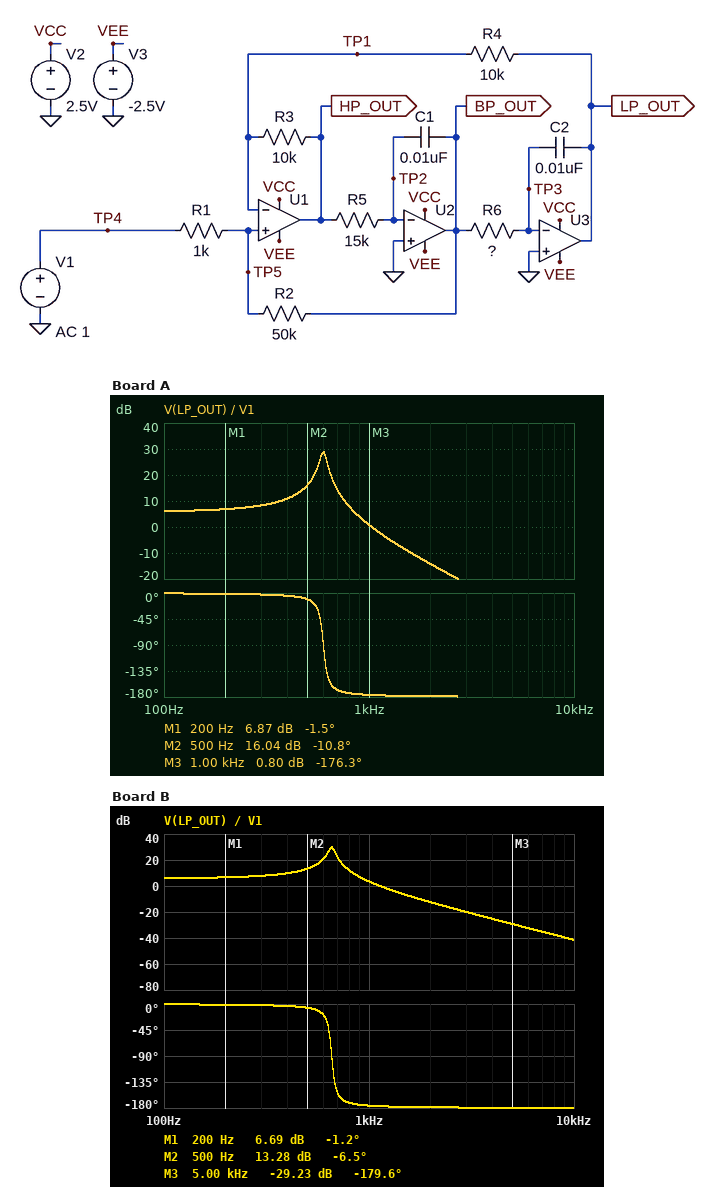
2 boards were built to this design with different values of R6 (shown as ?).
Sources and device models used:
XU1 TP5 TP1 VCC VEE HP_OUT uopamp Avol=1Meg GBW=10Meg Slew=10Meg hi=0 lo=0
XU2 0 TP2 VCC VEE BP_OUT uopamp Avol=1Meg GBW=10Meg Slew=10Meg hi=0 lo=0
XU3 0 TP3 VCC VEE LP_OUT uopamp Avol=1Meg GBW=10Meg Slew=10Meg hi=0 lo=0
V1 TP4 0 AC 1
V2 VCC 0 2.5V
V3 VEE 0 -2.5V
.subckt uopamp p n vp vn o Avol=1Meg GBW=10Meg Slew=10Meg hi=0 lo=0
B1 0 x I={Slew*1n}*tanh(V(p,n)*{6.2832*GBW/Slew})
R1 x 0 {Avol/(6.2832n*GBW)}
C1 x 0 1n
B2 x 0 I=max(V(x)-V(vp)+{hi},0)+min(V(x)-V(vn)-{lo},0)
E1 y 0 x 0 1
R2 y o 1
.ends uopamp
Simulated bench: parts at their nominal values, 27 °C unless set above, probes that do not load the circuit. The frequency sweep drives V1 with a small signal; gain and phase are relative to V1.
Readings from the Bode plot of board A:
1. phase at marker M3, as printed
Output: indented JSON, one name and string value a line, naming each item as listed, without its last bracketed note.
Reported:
{
  "phase at marker M3, as printed": "-176.3 deg"
}
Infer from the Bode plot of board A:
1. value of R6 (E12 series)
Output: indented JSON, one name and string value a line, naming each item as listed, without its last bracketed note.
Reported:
{
  "value of R6": "47 kΩ"
}
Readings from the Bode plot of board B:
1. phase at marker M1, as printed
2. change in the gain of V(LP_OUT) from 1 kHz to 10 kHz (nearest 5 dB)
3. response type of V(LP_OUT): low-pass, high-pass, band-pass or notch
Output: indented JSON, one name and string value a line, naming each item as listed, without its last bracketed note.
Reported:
{
  "phase at marker M1, as printed": "-1.2 deg",
  "change in the gain of V(LP_OUT) from 1 kHz to 10 kHz": "-45 dB",
  "response type of V(LP_OUT): low-pass, high-pass, band-pass or notch": "low-pass"
}
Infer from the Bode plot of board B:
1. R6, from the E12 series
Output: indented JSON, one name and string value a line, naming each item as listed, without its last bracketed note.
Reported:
{
  "R6, from the E12 series": "39 kΩ"
}
